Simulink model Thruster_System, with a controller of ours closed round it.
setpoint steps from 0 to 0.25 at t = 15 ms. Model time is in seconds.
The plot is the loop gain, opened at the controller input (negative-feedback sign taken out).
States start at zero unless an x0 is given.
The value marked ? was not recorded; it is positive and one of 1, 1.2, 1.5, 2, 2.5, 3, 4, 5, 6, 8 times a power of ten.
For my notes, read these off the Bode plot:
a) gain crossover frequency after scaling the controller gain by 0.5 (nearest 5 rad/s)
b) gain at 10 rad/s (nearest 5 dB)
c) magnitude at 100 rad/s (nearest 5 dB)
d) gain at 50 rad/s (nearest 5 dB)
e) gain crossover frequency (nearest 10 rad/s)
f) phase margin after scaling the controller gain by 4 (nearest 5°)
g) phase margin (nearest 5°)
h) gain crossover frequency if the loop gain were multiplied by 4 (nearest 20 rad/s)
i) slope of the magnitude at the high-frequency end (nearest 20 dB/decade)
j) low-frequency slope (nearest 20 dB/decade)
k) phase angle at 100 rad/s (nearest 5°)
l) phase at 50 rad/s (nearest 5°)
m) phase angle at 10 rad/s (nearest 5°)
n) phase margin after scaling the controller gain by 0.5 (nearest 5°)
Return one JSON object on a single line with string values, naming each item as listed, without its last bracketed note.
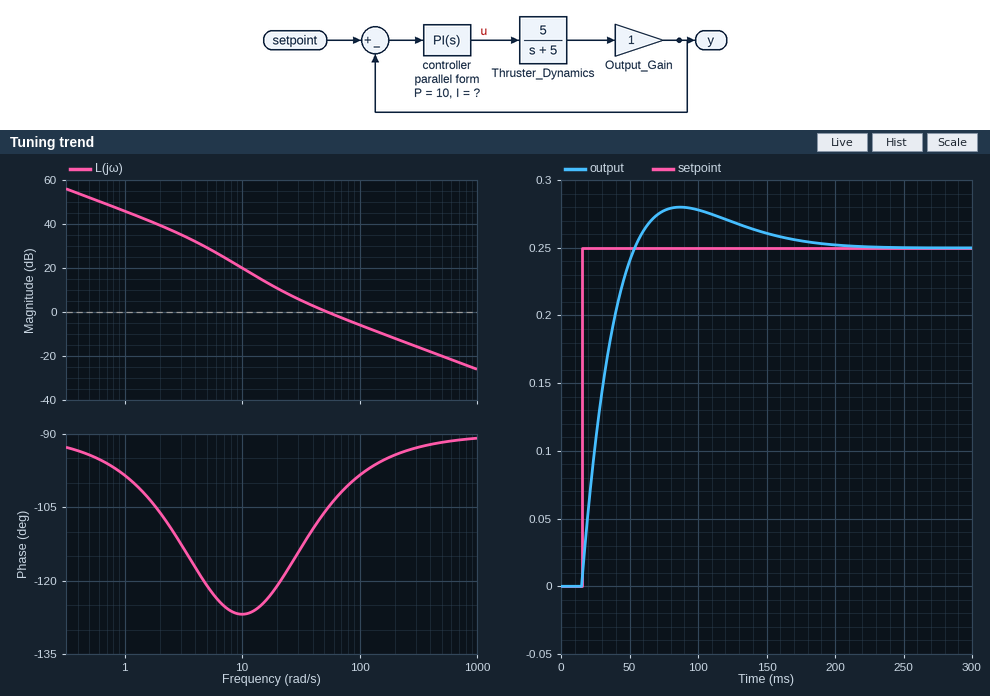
{"gain crossover frequency after scaling the controller gain by 0.5": "30 rad/s", "gain at 10 rad/s": "20 dB", "magnitude at 100 rad/s": "-5 dB", "gain at 50 rad/s": "0 dB", "gain crossover frequency": "50 rad/s", "phase margin after scaling the controller gain by 4": "85°", "phase margin": "75°", "gain crossover frequency if the loop gain were multiplied by 4": "200 rad/s", "slope of the magnitude at the high-frequency end": "-20 dB/decade", "low-frequency slope": "-20 dB/decade", "phase angle at 100 rad/s": "-100°", "phase at 50 rad/s": "-105°", "phase angle at 10 rad/s": "-125°", "phase margin after scaling the controller gain by 0.5": "65°"}
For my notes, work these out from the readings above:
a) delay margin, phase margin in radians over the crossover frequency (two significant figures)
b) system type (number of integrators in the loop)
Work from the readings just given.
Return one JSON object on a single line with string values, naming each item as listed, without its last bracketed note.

{"delay margin, phase margin in radians over the crossover frequency": "0.026 s", "system type": "1"}
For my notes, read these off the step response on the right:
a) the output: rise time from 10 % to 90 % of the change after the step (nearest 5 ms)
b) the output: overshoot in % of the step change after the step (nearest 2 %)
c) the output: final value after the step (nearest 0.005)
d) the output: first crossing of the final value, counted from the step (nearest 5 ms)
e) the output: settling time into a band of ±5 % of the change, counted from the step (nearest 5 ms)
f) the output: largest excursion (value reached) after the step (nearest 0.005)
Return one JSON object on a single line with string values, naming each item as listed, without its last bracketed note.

{"the output: rise time from 10 % to 90 % of the change after the step": "30 ms", "the output: overshoot in % of the step change after the step": "12 %", "the output: final value after the step": "0.250", "the output: first crossing of the final value, counted from the step": "40 ms", "the output: settling time into a band of ±5 % of the change, counted from the step": "130 ms", "the output: largest excursion (value reached) after the step": "0.280"}
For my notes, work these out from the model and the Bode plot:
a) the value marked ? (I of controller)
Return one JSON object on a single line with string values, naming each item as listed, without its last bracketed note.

{"the value marked ?": "200"}
